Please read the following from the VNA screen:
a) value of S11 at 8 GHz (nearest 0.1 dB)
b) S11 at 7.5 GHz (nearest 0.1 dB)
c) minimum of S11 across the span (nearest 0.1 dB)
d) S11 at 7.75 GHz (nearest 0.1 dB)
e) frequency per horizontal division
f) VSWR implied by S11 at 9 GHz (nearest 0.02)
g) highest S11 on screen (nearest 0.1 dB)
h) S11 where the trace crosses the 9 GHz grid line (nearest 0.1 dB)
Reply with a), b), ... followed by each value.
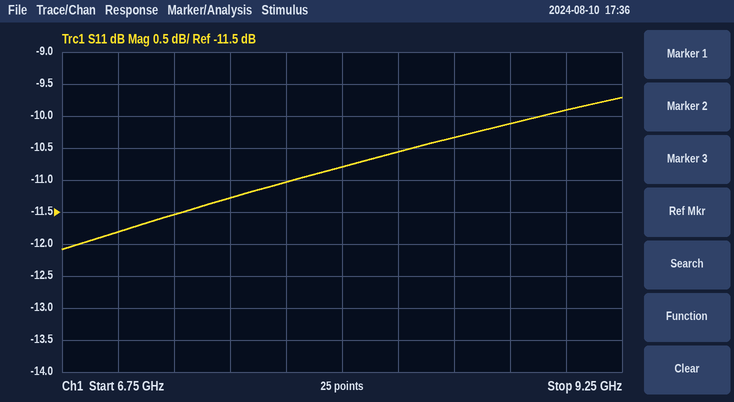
a) -10.8 dB
b) -11.3 dB
c) -12.1 dB
d) -11.0 dB
e) 250 MHz
f) 1.94
g) -9.7 dB
h) -9.9 dB
